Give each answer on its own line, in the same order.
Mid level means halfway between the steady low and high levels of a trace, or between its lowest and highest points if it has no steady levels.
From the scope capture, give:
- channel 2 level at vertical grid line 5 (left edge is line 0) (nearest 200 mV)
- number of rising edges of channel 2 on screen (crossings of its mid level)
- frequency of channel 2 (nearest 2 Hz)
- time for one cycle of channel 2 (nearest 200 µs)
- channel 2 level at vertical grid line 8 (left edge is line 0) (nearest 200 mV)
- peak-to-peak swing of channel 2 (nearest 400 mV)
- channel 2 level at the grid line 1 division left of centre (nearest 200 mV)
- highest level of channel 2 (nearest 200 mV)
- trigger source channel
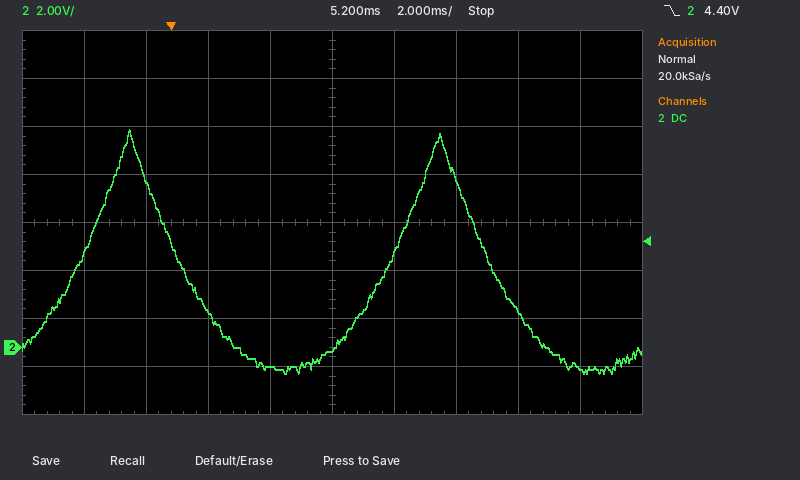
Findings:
0.0 V
2
100 Hz
10.0 ms
1.6 V
10.0 V
-800 mV
9.0 V
channel 2
